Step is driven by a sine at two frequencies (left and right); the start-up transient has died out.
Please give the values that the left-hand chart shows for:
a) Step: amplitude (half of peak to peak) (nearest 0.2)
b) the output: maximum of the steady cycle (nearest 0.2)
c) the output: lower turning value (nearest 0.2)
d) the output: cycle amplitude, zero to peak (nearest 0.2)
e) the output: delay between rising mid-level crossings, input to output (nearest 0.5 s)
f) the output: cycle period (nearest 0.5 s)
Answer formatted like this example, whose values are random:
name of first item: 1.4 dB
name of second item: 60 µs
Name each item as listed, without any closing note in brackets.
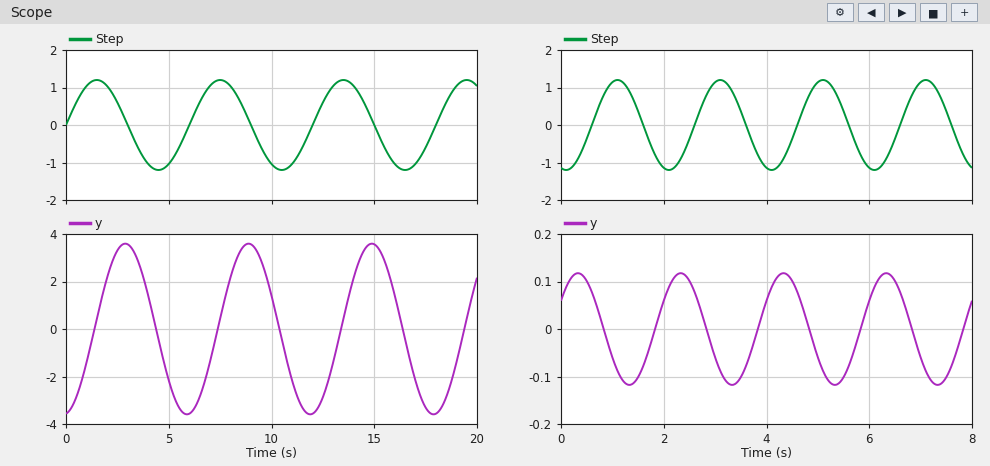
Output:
Step: amplitude (half of peak to peak): 1.2
the output: maximum of the steady cycle: 3.6
the output: lower turning value: -3.6
the output: cycle amplitude, zero to peak: 3.6
the output: delay between rising mid-level crossings, input to output: 1.5 s
the output: cycle period: 6.0 s
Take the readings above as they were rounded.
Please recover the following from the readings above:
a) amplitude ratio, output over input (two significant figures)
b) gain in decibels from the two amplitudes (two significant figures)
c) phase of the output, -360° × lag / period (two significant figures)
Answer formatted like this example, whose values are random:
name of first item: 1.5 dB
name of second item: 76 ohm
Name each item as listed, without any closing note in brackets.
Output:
amplitude ratio, output over input: 3.0
gain in decibels from the two amplitudes: 9.5 dB
phase of the output, -360° × lag / period: -90°
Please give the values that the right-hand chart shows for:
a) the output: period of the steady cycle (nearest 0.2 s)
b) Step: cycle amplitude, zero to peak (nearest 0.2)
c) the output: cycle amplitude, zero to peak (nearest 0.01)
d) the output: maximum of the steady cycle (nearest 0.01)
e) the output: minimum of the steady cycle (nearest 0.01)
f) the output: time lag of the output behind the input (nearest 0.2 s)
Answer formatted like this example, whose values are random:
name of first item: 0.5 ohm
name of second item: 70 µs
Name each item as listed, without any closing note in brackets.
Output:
the output: period of the steady cycle: 2.0 s
Step: cycle amplitude, zero to peak: 1.2
the output: cycle amplitude, zero to peak: 0.12
the output: maximum of the steady cycle: 0.12
the output: minimum of the steady cycle: -0.12
the output: time lag of the output behind the input: 1.2 s
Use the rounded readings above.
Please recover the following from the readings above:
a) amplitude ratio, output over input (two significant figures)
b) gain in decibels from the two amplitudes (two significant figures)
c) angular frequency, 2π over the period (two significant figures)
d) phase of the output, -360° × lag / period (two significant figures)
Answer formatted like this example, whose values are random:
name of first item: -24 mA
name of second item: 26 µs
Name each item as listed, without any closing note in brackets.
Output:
amplitude ratio, output over input: 0.10
gain in decibels from the two amplitudes: -20 dB
angular frequency, 2π over the period: 3.1 rad/s
phase of the output, -360° × lag / period: -220°
